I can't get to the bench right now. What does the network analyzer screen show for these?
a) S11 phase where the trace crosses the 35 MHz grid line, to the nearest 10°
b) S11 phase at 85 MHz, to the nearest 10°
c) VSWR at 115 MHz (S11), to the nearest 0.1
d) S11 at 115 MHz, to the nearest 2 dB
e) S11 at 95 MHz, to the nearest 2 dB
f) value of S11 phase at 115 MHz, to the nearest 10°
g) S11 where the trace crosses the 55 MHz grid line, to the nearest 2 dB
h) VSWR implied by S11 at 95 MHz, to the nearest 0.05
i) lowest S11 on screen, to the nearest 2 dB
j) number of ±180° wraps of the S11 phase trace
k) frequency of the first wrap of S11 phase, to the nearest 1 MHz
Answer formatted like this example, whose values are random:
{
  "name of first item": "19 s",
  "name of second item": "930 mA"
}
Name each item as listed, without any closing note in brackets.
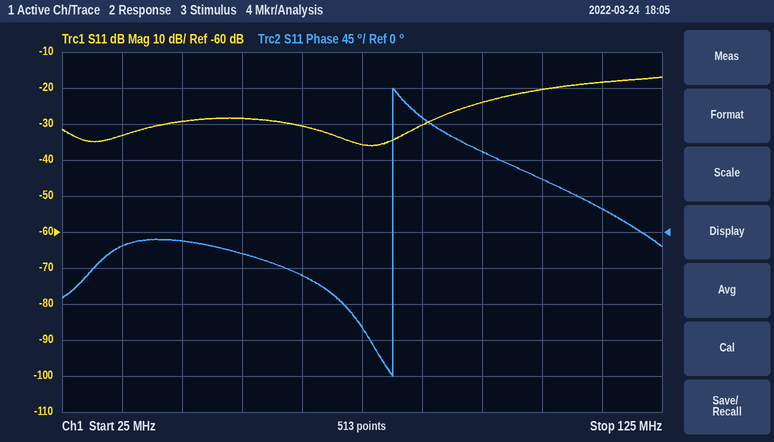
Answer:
{
  "S11 phase where the trace crosses the 35 MHz grid line, to the nearest 10°": "-20°",
  "S11 phase at 85 MHz, to the nearest 10°": "140°",
  "VSWR at 115 MHz (S11), to the nearest 0.1": "1.3",
  "S11 at 115 MHz, to the nearest 2 dB": "-18 dB",
  "S11 at 95 MHz, to the nearest 2 dB": "-24 dB",
  "value of S11 phase at 115 MHz, to the nearest 10°": "30°",
  "S11 where the trace crosses the 55 MHz grid line, to the nearest 2 dB": "-28 dB",
  "VSWR implied by S11 at 95 MHz, to the nearest 0.05": "1.15",
  "lowest S11 on screen, to the nearest 2 dB": "-36 dB",
  "number of ±180° wraps of the S11 phase trace": "1",
  "frequency of the first wrap of S11 phase, to the nearest 1 MHz": "80 MHz"
}
